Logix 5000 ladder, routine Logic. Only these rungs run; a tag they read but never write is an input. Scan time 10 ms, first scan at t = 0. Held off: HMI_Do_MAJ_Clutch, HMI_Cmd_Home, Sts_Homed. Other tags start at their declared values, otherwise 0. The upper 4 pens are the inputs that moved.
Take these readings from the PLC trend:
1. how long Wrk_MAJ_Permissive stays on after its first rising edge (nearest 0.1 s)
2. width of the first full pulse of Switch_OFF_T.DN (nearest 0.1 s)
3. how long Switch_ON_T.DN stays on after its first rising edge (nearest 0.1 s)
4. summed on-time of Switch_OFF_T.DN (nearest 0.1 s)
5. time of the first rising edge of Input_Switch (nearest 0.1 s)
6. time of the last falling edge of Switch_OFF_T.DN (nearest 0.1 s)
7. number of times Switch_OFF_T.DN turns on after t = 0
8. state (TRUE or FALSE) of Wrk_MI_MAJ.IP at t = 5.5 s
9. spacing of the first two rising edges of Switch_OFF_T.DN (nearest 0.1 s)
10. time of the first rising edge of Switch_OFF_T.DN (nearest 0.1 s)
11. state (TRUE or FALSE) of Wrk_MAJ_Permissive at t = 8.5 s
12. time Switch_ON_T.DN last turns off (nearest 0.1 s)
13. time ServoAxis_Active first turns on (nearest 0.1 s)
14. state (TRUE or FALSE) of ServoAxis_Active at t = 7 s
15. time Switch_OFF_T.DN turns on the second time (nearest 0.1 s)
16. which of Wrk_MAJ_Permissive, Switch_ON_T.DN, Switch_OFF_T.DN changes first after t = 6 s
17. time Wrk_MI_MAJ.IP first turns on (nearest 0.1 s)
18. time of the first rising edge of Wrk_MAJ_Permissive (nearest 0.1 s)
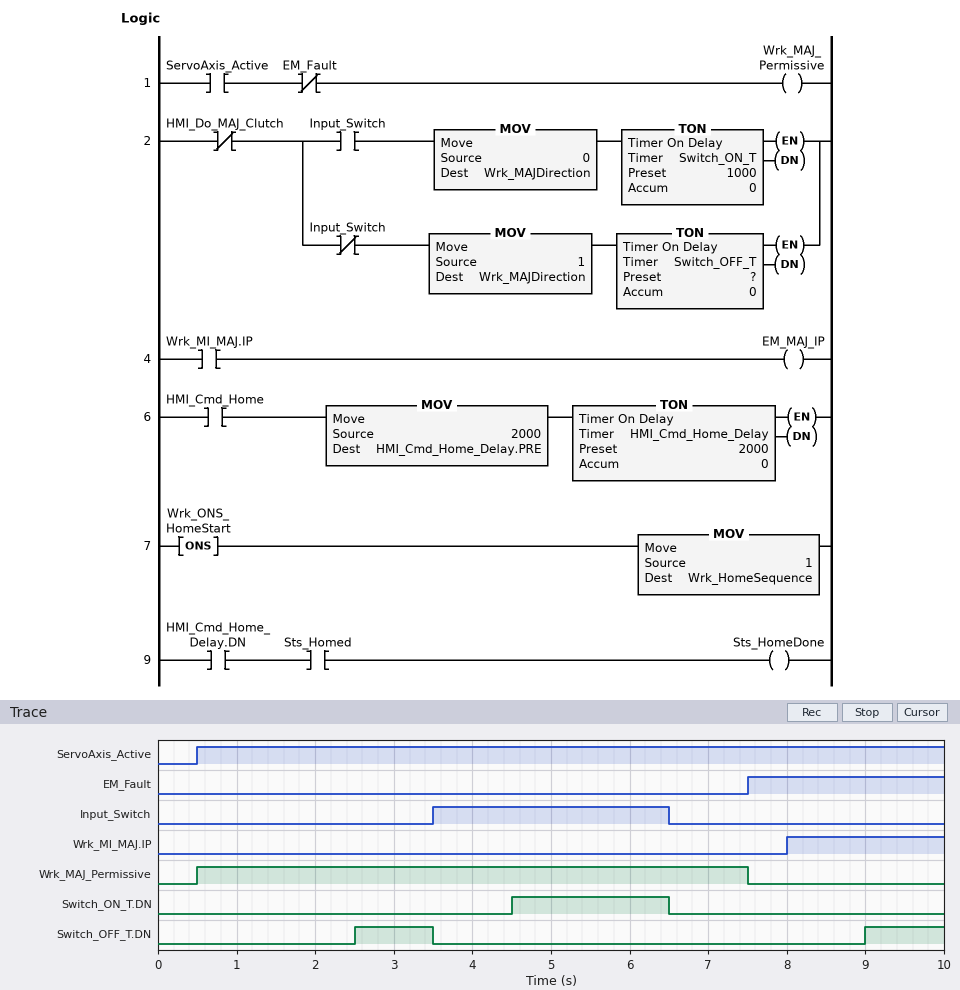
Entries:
7.0 s
1.0 s
2.0 s
2.0 s
3.5 s
3.5 s
2
FALSE
6.5 s
2.5 s
FALSE
6.5 s
0.5 s
TRUE
9.0 s
Switch_ON_T.DN
8.0 s
0.5 s
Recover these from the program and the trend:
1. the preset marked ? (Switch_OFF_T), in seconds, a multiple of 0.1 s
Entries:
2.5 s
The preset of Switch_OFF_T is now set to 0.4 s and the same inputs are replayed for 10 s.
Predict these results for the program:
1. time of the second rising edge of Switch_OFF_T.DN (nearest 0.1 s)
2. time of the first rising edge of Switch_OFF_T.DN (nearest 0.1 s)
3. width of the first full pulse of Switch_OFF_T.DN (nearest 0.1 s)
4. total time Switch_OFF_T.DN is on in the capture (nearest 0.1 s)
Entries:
6.9 s
0.4 s
3.1 s
6.2 s
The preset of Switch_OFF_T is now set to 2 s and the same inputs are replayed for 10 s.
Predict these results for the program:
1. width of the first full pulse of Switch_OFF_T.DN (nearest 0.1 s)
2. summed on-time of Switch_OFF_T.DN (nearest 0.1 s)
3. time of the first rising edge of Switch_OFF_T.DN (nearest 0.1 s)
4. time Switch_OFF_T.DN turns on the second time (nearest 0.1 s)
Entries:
1.5 s
3.0 s
2.0 s
8.5 s
